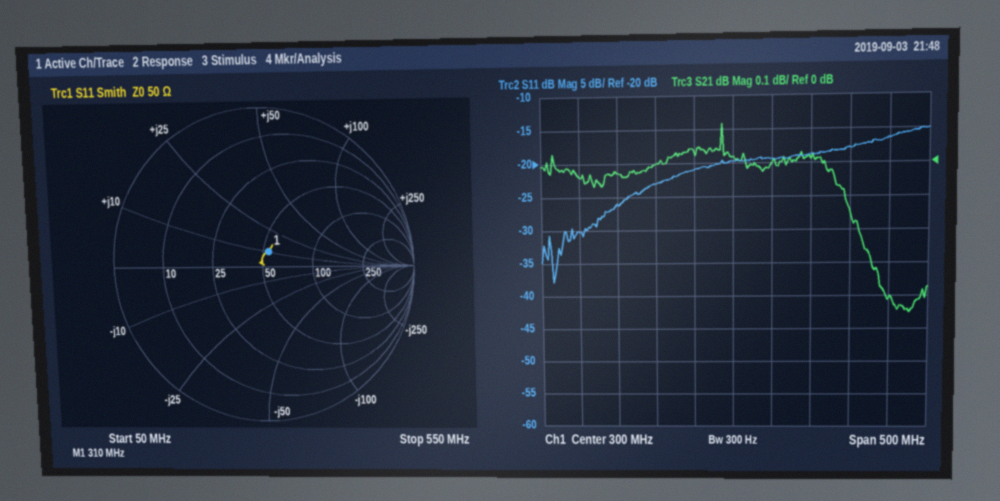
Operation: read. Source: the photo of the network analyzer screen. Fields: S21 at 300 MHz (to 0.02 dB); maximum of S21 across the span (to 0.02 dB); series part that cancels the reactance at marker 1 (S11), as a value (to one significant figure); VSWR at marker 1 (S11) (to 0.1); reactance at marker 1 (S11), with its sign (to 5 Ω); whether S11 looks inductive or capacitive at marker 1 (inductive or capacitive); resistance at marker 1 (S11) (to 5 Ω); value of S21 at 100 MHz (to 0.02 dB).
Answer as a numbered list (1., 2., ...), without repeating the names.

1. 0.02 dB
2. 0.12 dB
3. 50 pF
4. 1.2
5. +10 Ω
6. inductive
7. 55 Ω
8. -0.04 dB
